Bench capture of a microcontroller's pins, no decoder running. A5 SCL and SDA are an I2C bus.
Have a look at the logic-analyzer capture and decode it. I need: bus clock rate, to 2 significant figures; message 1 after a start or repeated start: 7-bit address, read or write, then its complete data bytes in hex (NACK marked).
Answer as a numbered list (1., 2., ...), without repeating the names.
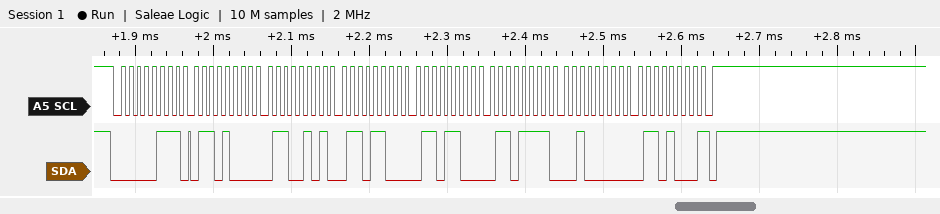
1. 100 kHz
2. 0x03 read: 68 65 6C 6C 6F 20 68 NACK
